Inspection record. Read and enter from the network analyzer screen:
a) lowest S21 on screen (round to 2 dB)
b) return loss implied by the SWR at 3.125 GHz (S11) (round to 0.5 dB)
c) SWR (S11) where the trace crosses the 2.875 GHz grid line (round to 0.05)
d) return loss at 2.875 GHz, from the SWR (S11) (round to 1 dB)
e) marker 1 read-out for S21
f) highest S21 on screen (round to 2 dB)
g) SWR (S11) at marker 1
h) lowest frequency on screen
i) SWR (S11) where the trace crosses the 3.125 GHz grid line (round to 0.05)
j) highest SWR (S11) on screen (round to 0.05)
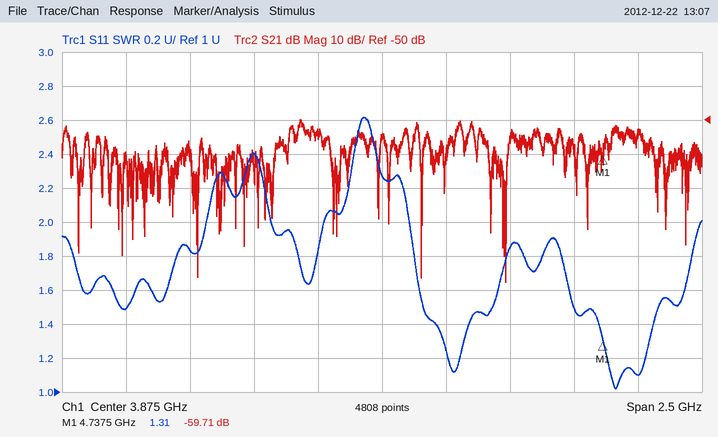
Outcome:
-98 dB
10.5 dB
1.50
14 dB
-59.71 dB
-50 dB
1.31
2.625 GHz
1.85
2.60
